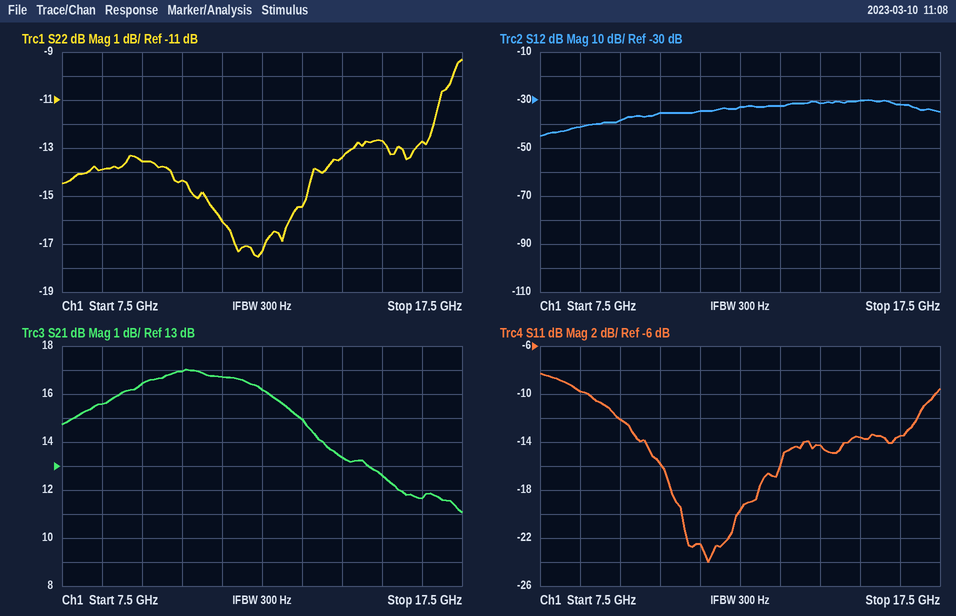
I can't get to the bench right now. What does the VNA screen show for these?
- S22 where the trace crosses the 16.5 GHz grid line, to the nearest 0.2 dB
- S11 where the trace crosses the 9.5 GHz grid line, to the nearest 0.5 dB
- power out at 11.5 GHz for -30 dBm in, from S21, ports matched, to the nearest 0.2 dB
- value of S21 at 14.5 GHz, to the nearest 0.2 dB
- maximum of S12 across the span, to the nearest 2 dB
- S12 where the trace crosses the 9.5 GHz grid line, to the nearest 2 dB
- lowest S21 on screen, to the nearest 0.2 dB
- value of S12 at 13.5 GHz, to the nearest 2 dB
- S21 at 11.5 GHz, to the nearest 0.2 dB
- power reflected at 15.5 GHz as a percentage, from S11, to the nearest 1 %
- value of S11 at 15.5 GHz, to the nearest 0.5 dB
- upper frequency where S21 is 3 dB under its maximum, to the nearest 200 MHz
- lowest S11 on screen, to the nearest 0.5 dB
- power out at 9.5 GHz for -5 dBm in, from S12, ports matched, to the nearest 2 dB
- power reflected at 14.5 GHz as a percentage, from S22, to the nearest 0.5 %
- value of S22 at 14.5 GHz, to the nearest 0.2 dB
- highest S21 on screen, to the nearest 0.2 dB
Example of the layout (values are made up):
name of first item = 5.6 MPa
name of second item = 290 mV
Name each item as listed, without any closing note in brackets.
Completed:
S22 where the trace crosses the 16.5 GHz grid line, to the nearest 0.2 dB = -12.8 dB
S11 where the trace crosses the 9.5 GHz grid line, to the nearest 0.5 dB = -12.0 dB
power out at 11.5 GHz for -30 dBm in, from S21, ports matched, to the nearest 0.2 dB = -13.2 dBm
value of S21 at 14.5 GHz, to the nearest 0.2 dB = 13.4 dB
maximum of S12 across the span, to the nearest 2 dB = -30 dB
S12 where the trace crosses the 9.5 GHz grid line, to the nearest 2 dB = -38 dB
lowest S21 on screen, to the nearest 0.2 dB = 11.0 dB
value of S12 at 13.5 GHz, to the nearest 2 dB = -32 dB
S21 at 11.5 GHz, to the nearest 0.2 dB = 16.8 dB
power reflected at 15.5 GHz as a percentage, from S11, to the nearest 1 % = 4 %
value of S11 at 15.5 GHz, to the nearest 0.5 dB = -13.5 dB
upper frequency where S21 is 3 dB under its maximum, to the nearest 200 MHz = 14.0 GHz
lowest S11 on screen, to the nearest 0.5 dB = -24.0 dB
power out at 9.5 GHz for -5 dBm in, from S12, ports matched, to the nearest 2 dB = -44 dBm
power reflected at 14.5 GHz as a percentage, from S22, to the nearest 0.5 % = 4.5 %
value of S22 at 14.5 GHz, to the nearest 0.2 dB = -13.4 dB
highest S21 on screen, to the nearest 0.2 dB = 17.0 dB
